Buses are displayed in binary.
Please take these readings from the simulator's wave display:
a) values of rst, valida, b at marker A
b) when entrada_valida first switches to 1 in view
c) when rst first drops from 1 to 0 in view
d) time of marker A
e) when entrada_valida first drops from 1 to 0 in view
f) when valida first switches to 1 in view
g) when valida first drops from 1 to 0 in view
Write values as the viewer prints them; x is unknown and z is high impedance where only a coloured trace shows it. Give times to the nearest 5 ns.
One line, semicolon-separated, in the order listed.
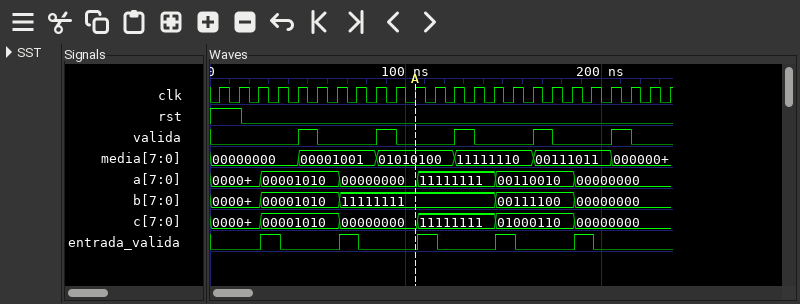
rst=0, valida=0, b=11111111; 25 ns; 15 ns; 105 ns; 35 ns; 45 ns; 55 ns
